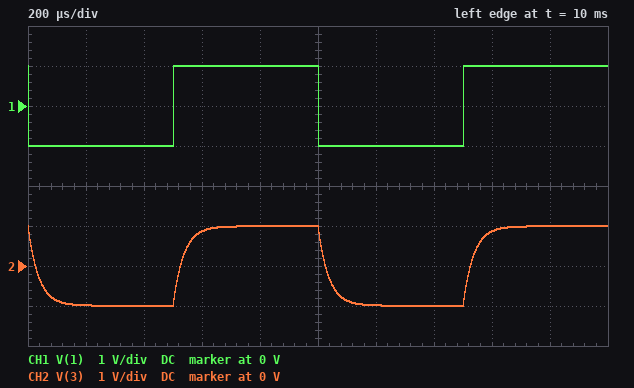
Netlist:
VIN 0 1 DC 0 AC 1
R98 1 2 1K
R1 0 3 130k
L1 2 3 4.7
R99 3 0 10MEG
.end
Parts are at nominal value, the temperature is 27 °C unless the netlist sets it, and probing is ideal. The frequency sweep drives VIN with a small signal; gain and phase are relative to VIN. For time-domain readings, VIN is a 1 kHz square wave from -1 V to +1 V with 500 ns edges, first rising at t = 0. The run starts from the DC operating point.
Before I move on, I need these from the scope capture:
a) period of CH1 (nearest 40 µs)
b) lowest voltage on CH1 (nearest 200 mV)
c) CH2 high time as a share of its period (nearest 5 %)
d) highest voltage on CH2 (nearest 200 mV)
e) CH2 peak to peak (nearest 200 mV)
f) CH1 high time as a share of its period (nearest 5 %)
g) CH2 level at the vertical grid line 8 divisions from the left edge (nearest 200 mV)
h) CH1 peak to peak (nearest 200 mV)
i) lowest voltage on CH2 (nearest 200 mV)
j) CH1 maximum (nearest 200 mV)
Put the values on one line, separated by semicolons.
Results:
1.00 ms; -1.0 V; 50 %; 1.0 V; 2.0 V; 50 %; 800 mV; 2.0 V; -1.0 V; 1.0 V
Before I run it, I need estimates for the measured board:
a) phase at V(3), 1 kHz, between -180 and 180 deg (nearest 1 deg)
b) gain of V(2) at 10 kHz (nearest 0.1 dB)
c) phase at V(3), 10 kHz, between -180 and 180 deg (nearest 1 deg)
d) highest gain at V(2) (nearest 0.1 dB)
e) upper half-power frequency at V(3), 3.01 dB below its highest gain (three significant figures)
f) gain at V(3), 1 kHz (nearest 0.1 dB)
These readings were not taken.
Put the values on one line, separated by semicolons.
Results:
167 deg; 0 dB; 114 deg; 0 dB; 4.38 kHz; -0.3 dB
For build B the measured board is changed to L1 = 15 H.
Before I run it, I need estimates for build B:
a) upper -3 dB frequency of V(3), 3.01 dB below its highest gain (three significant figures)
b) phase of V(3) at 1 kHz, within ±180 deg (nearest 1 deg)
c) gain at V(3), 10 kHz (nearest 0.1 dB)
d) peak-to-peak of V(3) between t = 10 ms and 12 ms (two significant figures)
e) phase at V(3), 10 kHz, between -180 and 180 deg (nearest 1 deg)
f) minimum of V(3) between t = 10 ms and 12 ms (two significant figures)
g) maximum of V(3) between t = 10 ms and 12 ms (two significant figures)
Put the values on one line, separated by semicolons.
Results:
1.37 kHz; 144 deg; -17.4 dB; 1.9 V; 98 deg; -970 mV; 970 mV
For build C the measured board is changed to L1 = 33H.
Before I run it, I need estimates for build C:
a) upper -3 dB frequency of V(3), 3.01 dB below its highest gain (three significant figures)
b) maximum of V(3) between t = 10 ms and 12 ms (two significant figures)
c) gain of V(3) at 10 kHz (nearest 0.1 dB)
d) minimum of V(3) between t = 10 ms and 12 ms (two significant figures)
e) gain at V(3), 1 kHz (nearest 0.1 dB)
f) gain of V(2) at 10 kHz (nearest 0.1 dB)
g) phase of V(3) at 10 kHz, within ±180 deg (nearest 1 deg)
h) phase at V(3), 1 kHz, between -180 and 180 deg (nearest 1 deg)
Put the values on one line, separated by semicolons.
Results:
624 Hz; 750 mV; -24.2 dB; -750 mV; -5.6 dB; 0 dB; 94 deg; 122 deg
